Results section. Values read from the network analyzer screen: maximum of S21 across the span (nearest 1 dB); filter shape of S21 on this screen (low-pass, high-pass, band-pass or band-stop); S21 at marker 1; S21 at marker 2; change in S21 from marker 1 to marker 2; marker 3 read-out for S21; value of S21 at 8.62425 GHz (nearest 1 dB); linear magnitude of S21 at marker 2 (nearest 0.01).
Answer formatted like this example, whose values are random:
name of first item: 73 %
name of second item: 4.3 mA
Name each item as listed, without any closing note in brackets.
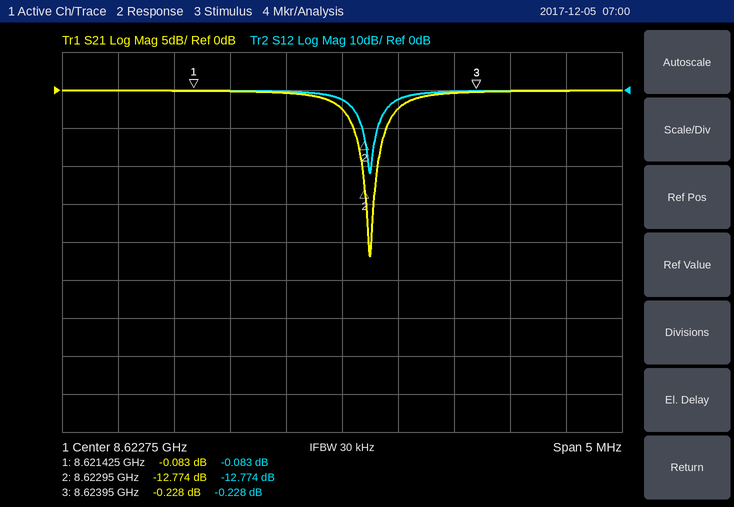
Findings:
maximum of S21 across the span: 0 dB
filter shape of S21 on this screen: band-stop
S21 at marker 1: -0.083 dB
S21 at marker 2: -12.774 dB
change in S21 from marker 1 to marker 2: -12.691 dB
marker 3 read-out for S21: -0.228 dB
value of S21 at 8.62425 GHz: 0 dB
linear magnitude of S21 at marker 2: 0.23
